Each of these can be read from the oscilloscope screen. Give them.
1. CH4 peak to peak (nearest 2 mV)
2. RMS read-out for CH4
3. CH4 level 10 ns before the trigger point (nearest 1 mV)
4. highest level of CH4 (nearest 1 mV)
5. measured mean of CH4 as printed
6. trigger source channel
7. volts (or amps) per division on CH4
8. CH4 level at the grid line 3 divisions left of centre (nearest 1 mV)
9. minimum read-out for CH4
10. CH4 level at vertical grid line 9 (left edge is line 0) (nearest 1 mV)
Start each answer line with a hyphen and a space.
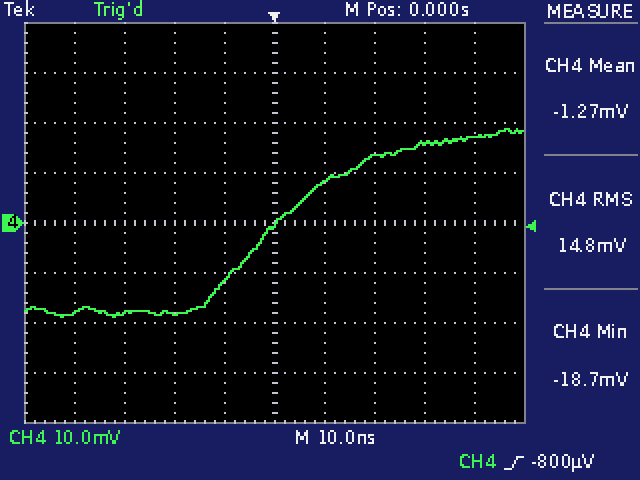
- 38 mV
- 14.8 mV
- -12 mV
- 19 mV
- -1.27 mV
- CH4
- 10 mV
- -18 mV
- -18.7 mV
- 17 mV
